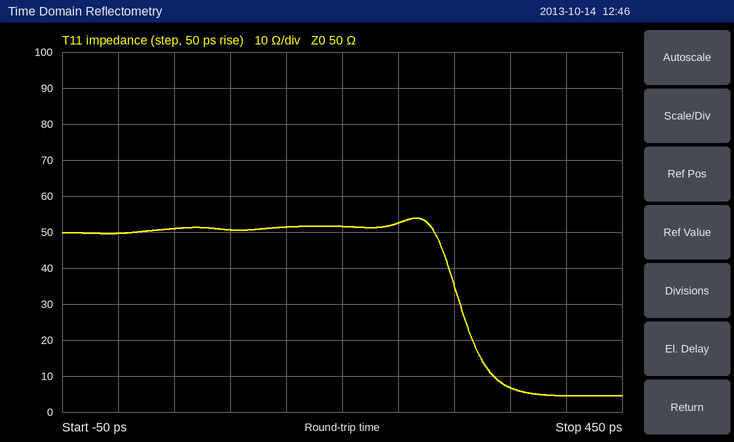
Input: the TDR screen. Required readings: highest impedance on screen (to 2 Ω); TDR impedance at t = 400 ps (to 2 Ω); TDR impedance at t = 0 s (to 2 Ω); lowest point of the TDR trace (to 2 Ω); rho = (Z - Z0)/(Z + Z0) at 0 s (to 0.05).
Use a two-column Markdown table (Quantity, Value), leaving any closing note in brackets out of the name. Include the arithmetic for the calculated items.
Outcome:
| Quantity | Value |
|---|---|
| highest impedance on screen | 54 Ω |
| TDR impedance at t = 400 ps | 4 Ω |
| TDR impedance at t = 0 s | 50 Ω |
| lowest point of the TDR trace | 4 Ω |
| rho = (Z - Z0)/(Z + Z0) at 0 s | (50 − 50)/(50 + 50) ≈ 0.00 |
